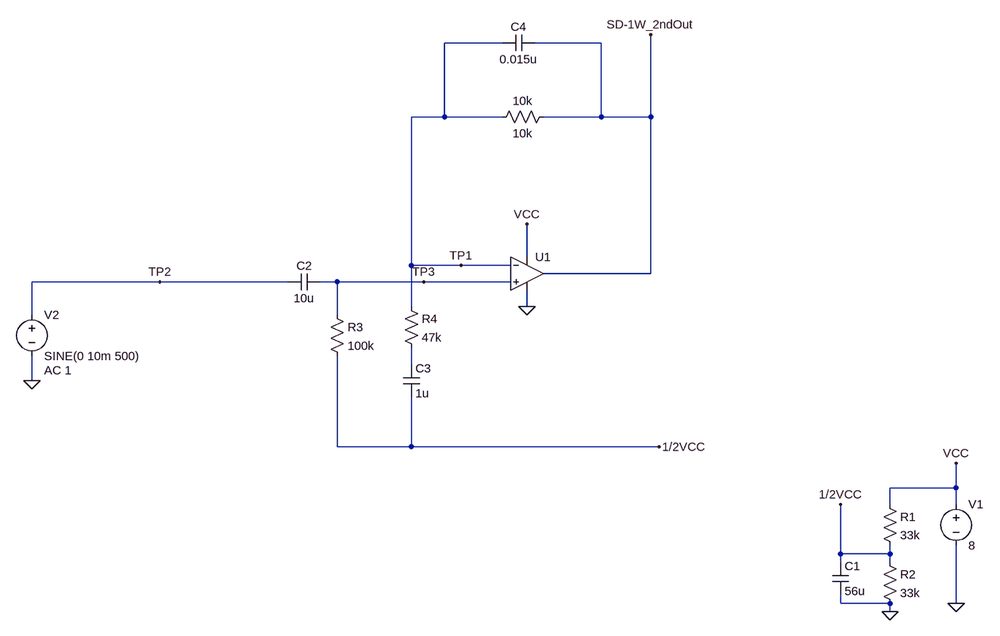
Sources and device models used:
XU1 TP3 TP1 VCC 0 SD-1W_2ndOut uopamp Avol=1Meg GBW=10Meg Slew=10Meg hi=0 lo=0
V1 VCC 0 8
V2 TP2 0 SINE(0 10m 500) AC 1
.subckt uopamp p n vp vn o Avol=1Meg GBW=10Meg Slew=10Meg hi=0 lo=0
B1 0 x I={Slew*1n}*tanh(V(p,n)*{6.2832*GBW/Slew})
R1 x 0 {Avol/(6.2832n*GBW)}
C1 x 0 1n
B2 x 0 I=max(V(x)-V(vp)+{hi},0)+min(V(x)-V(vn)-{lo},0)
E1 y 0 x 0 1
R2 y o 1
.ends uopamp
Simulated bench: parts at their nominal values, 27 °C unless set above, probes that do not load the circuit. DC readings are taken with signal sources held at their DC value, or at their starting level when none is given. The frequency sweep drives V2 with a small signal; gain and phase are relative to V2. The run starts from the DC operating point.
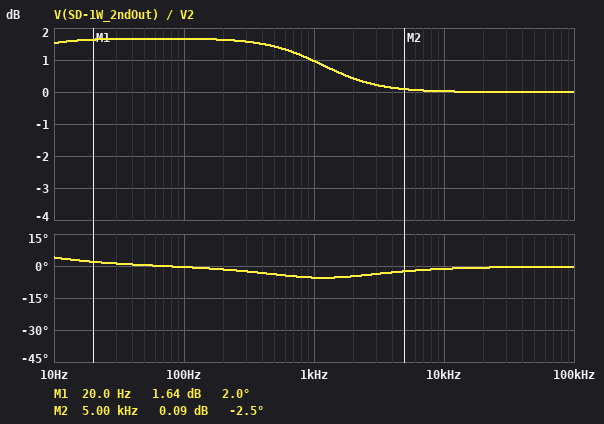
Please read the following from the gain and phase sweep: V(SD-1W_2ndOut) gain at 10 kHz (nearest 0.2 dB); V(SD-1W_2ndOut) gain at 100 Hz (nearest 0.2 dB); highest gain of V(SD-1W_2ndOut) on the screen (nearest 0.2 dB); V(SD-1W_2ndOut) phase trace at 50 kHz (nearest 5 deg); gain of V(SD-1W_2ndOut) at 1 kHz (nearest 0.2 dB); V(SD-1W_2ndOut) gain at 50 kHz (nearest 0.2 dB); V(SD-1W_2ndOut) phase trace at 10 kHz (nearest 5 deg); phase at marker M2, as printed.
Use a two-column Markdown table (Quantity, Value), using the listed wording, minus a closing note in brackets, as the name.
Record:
| Quantity | Value |
|---|---|
| V(SD-1W_2ndOut) gain at 10 kHz | 0 dB |
| V(SD-1W_2ndOut) gain at 100 Hz | 1.6 dB |
| highest gain of V(SD-1W_2ndOut) on the screen | 1.6 dB |
| V(SD-1W_2ndOut) phase trace at 50 kHz | 0 deg |
| gain of V(SD-1W_2ndOut) at 1 kHz | 1.0 dB |
| V(SD-1W_2ndOut) gain at 50 kHz | 0 dB |
| V(SD-1W_2ndOut) phase trace at 10 kHz | 0 deg |
| phase at marker M2, as printed | -2.5 deg |
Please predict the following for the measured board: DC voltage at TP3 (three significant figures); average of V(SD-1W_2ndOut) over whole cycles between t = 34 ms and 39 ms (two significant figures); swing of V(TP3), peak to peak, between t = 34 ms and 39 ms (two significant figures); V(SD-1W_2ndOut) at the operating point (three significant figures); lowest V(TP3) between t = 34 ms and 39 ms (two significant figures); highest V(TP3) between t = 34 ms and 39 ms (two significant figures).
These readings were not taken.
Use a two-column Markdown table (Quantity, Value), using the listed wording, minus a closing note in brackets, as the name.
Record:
| Quantity | Value |
|---|---|
| DC voltage at TP3 | 4.00 V |
| average of V(SD-1W_2ndOut) over whole cycles between t = 34 ms and 39 ms | 4.0 V |
| swing of V(TP3), peak to peak, between t = 34 ms and 39 ms | 20 mV |
| V(SD-1W_2ndOut) at the operating point | 4.00 V |
| lowest V(TP3) between t = 34 ms and 39 ms | 4.0 V |
| highest V(TP3) between t = 34 ms and 39 ms | 4.0 V |
